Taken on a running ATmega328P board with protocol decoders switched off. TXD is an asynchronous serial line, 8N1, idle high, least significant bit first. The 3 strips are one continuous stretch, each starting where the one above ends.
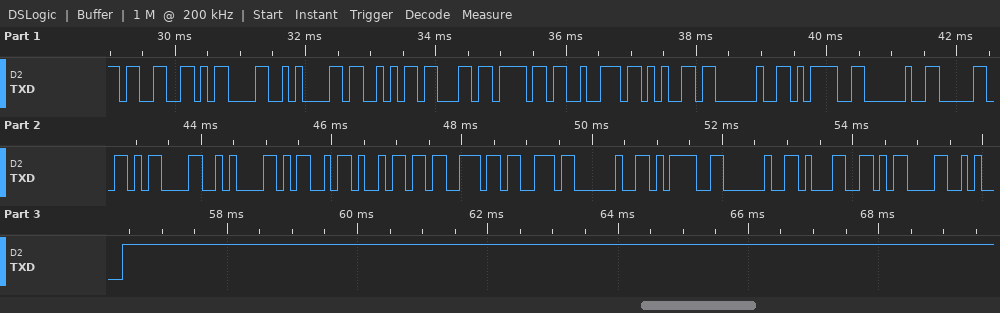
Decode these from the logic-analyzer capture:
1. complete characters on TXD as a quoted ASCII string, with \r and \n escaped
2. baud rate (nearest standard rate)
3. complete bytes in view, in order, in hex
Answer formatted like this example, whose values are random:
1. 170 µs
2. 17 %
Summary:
1. "3\r\nScore = 0\r\nMiss = 1\r\n"
2. 9600 baud
3. 33 0D 0A 53 63 6F 72 65 20 3D 20 30 0D 0A 4D 69 73 73 20 3D 20 31 0D 0A
